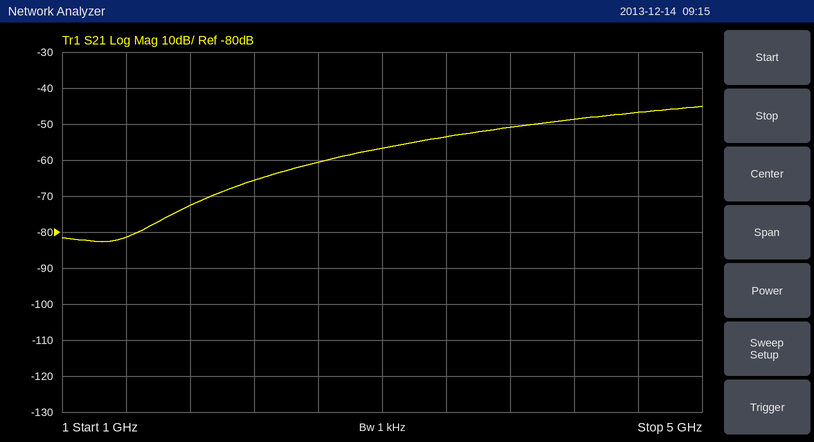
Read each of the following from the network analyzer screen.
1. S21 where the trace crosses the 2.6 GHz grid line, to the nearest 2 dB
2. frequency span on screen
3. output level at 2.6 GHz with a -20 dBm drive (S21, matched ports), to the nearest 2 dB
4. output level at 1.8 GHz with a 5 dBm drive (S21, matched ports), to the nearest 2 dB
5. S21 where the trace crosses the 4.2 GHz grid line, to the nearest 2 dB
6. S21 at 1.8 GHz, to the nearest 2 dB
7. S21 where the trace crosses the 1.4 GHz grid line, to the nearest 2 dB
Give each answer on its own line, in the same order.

-60 dB
4 GHz
-80 dBm
-68 dBm
-48 dB
-72 dB
-82 dB
